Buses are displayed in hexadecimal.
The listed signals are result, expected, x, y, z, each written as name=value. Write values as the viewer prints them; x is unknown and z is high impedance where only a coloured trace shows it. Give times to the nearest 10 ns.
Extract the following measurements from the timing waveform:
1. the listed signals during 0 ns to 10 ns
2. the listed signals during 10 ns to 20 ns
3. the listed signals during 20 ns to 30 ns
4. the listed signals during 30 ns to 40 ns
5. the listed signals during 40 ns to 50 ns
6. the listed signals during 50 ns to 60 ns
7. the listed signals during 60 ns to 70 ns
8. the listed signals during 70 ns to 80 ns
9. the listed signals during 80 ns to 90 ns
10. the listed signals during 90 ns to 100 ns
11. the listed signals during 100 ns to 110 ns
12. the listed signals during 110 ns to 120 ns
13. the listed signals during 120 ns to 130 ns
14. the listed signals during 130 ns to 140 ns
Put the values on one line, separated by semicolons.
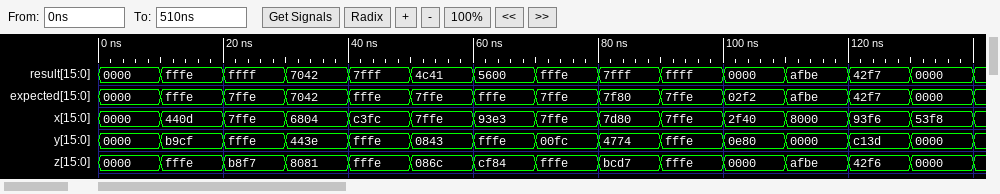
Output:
result=0000, expected=0000, x=0000, y=0000, z=0000; result=fffe, expected=fffe, x=440d, y=b9cf, z=fffe; result=ffff, expected=7ffe, x=7ffe, y=fffe, z=b8f7; result=7042, expected=7042, x=6804, y=443e, z=8081; result=7fff, expected=fffe, x=c3fc, y=fffe, z=fffe; result=4c41, expected=7ffe, x=7ffe, y=0843, z=086c; result=5600, expected=fffe, x=93e3, y=fffe, z=cf84; result=fffe, expected=7ffe, x=7ffe, y=00fc, z=fffe; result=7fff, expected=7f80, x=7d80, y=4774, z=bcd7; result=ffff, expected=7ffe, x=7ffe, y=fffe, z=fffe; result=0000, expected=02f2, x=2f40, y=0e80, z=0000; result=afbe, expected=afbe, x=8000, y=0000, z=afbe; result=42f7, expected=42f7, x=93f6, y=c13d, z=42f6; result=0000, expected=0000, x=53f8, y=0000, z=0000
